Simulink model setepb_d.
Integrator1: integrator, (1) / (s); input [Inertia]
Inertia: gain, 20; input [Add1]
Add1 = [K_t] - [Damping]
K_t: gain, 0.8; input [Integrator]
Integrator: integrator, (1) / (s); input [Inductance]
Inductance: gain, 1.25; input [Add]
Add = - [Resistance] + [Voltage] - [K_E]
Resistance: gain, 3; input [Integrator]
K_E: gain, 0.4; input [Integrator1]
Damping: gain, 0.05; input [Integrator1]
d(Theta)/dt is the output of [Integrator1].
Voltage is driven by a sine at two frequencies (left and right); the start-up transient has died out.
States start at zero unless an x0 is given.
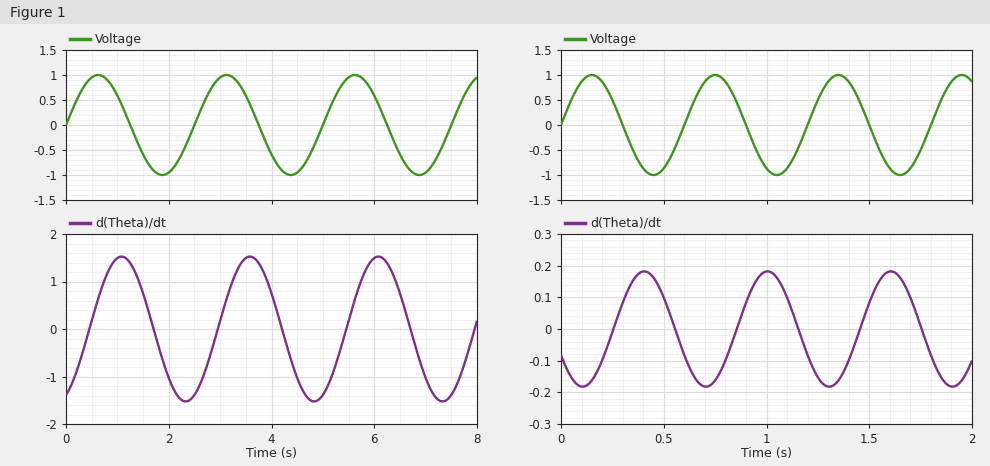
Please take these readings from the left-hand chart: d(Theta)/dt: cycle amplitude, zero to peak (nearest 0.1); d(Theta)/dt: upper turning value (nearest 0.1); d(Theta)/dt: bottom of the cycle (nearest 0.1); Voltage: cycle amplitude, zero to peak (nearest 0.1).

1.5
1.5
-1.5
1.0
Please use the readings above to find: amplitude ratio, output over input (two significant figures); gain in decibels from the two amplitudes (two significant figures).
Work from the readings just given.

1.5
3.5 dB
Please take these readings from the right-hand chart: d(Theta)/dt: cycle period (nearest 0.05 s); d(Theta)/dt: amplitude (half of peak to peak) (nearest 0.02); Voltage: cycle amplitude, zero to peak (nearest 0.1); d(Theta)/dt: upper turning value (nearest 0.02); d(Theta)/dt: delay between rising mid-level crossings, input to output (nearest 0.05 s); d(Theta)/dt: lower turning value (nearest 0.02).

0.60 s
0.18
1.0
0.18
0.25 s
-0.18
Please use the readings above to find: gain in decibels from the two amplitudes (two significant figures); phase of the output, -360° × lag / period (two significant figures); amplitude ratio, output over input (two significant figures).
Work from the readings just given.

-15 dB
-150°
0.18
